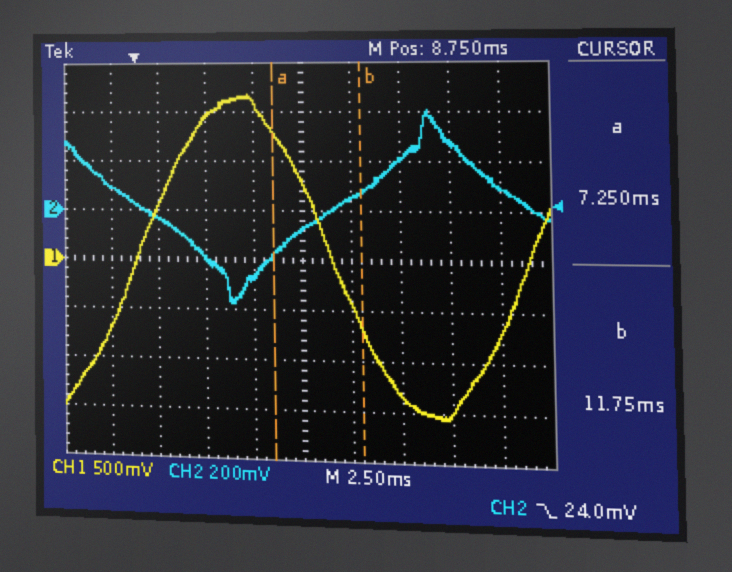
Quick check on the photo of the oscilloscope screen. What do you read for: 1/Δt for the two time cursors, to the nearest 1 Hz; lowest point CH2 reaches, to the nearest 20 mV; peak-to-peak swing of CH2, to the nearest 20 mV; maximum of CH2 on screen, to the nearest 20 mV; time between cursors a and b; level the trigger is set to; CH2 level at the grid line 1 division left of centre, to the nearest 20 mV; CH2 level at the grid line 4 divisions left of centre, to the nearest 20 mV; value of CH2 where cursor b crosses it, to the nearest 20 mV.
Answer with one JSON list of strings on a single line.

["222 Hz", "-380 mV", "780 mV", "400 mV", "4.50 ms", "24.0 mV", "-260 mV", "100 mV", "80 mV"]
